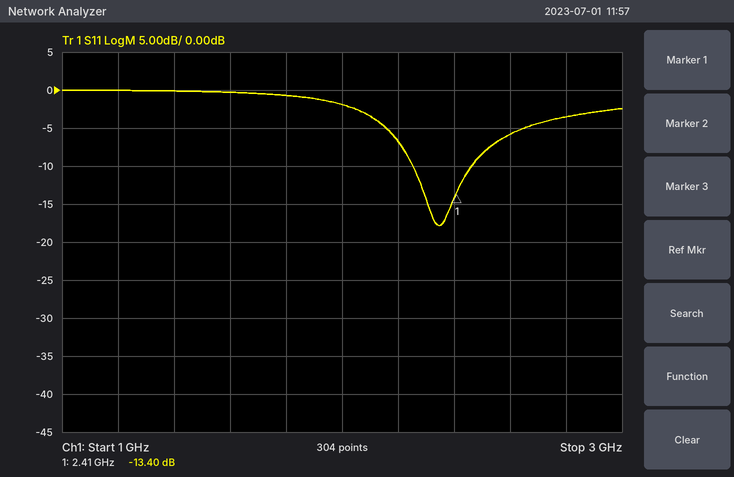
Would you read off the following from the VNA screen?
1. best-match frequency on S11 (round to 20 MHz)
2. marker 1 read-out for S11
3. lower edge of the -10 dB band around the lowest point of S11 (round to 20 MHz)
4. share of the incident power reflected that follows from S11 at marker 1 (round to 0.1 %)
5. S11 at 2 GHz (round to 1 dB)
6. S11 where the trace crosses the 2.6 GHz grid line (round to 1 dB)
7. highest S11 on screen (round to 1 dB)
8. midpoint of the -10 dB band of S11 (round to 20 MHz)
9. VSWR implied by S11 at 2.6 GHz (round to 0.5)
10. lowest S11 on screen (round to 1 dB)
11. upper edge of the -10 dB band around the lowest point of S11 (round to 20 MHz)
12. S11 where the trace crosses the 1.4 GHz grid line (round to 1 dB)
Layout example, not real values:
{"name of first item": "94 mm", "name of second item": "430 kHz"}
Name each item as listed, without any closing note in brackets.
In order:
{"best-match frequency on S11": "2.34 GHz", "marker 1 read-out for S11": "-13.40 dB", "lower edge of the -10 dB band around the lowest point of S11": "2.26 GHz", "share of the incident power reflected that follows from S11 at marker 1": "4.6 %", "S11 at 2 GHz": "-2 dB", "S11 where the trace crosses the 2.6 GHz grid line": "-6 dB", "highest S11 on screen": "0 dB", "midpoint of the -10 dB band of S11": "2.36 GHz", "VSWR implied by S11 at 2.6 GHz": "3.0", "lowest S11 on screen": "-18 dB", "upper edge of the -10 dB band around the lowest point of S11": "2.46 GHz", "S11 where the trace crosses the 1.4 GHz grid line": "0 dB"}
